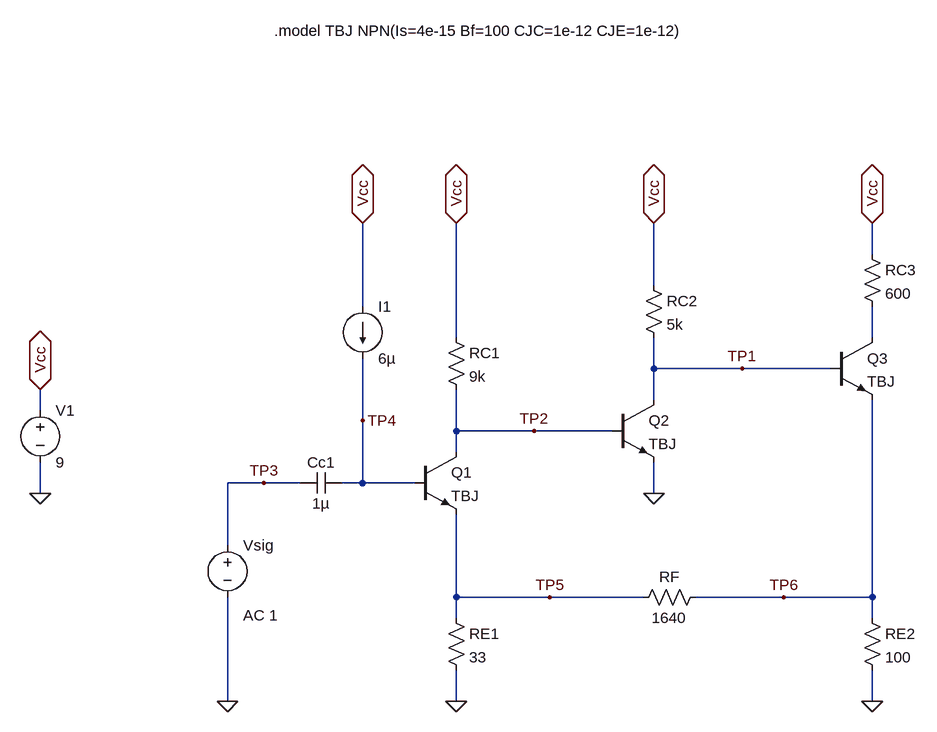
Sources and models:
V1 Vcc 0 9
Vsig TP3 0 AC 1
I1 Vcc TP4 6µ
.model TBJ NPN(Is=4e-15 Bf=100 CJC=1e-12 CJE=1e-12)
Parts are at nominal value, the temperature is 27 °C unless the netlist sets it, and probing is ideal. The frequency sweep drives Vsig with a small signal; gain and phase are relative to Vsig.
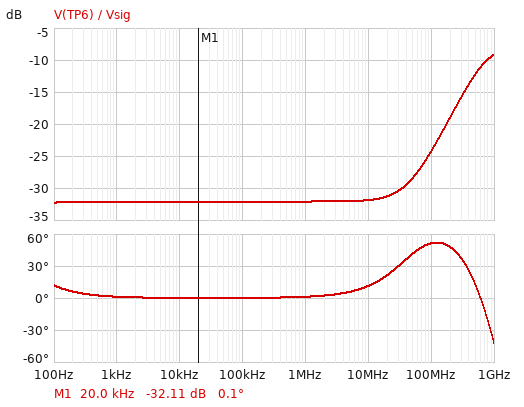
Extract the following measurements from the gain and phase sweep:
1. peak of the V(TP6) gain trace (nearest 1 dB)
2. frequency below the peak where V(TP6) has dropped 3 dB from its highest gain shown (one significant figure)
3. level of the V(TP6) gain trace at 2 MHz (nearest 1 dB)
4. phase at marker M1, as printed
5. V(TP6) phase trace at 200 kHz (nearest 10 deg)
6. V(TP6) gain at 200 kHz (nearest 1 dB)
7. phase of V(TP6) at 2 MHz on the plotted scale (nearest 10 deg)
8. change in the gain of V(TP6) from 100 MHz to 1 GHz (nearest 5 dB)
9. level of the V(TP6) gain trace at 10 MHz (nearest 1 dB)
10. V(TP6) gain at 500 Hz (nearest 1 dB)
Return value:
-9 dB
500 MHz
-32 dB
0.1 deg
0 deg
-32 dB
0 deg
15 dB
-32 dB
-32 dB
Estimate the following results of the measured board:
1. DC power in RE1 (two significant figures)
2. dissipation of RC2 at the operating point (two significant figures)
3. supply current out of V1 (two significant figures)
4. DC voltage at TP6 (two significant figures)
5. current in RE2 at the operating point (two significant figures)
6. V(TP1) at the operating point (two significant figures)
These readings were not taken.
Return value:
12 µW
16 mW
2.7 mA
1.1 mV
11 µA
54 mV
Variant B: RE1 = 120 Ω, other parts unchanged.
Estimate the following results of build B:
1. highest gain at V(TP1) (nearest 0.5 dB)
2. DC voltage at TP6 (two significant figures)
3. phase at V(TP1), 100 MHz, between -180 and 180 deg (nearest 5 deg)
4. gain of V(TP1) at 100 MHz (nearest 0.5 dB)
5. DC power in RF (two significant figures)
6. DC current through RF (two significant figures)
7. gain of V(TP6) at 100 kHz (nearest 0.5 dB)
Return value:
-7.5 dB
3.9 mV
-15 deg
-8.0 dB
2.5 µW
39 µA
-27.5 dB
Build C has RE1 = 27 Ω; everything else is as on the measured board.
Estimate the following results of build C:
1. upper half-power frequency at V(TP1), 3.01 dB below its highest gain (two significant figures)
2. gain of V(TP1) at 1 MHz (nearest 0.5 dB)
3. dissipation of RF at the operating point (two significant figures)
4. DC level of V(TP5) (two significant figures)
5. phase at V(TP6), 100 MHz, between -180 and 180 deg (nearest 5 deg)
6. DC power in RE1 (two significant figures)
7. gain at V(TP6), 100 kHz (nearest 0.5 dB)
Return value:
1.1 GHz
-1.0 dB
140 nW
16 mV
55 deg
9.6 µW
-33.0 dB
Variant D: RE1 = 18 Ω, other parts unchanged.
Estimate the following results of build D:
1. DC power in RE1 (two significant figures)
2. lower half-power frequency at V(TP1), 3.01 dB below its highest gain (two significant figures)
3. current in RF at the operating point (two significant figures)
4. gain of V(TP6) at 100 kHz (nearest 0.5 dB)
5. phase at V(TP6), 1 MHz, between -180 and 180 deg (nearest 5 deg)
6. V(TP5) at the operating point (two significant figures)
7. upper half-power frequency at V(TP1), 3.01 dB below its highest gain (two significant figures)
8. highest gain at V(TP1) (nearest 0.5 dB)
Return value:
6.5 µW
26 Hz
6.2 µA
-35.5 dB
0 deg
11 mV
1.0 GHz
0.5 dB
